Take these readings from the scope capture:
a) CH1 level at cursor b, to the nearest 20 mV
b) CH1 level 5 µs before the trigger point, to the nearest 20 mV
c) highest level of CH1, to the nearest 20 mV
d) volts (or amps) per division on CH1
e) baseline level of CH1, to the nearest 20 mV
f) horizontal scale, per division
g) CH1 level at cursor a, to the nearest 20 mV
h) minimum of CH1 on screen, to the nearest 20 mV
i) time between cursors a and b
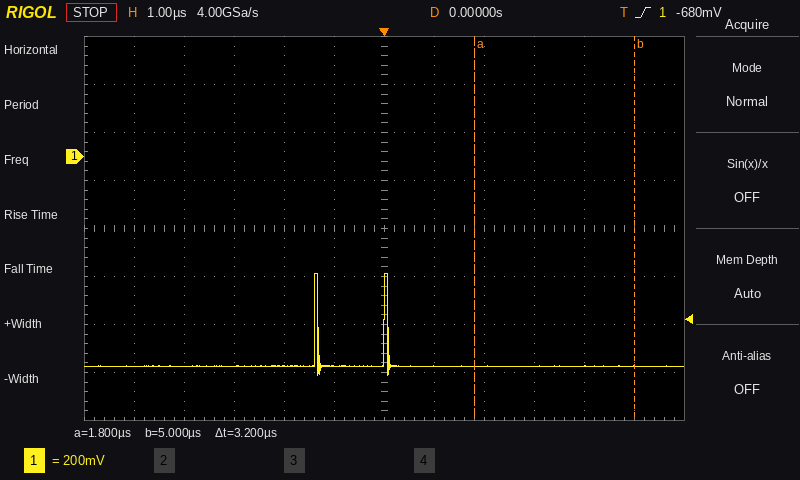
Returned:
-880 mV
-880 mV
-480 mV
200 mV
-880 mV
1 µs
-880 mV
-920 mV
3.2 µs
